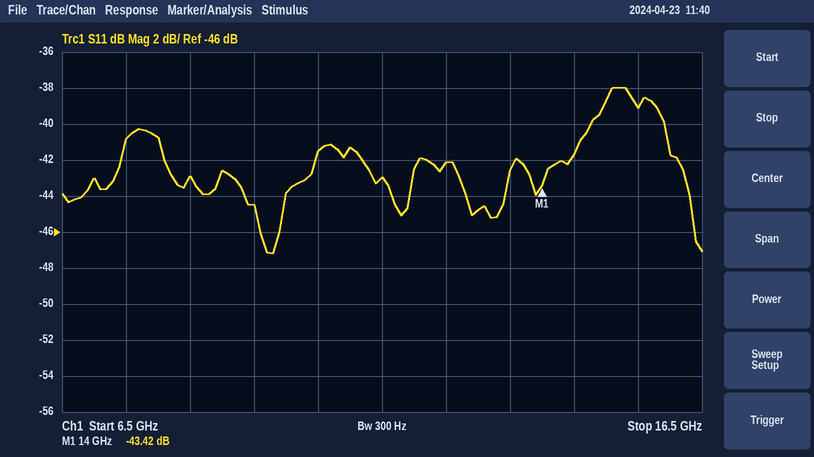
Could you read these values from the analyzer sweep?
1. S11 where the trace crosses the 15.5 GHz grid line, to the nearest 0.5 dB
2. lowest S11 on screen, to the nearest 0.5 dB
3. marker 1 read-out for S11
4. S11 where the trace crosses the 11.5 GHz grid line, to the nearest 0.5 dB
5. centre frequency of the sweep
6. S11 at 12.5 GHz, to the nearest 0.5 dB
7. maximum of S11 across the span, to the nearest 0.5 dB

-39.0 dB
-47.0 dB
-43.42 dB
-43.0 dB
11.5 GHz
-42.0 dB
-38.0 dB
